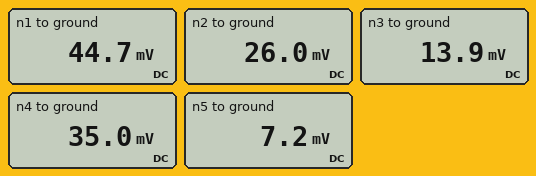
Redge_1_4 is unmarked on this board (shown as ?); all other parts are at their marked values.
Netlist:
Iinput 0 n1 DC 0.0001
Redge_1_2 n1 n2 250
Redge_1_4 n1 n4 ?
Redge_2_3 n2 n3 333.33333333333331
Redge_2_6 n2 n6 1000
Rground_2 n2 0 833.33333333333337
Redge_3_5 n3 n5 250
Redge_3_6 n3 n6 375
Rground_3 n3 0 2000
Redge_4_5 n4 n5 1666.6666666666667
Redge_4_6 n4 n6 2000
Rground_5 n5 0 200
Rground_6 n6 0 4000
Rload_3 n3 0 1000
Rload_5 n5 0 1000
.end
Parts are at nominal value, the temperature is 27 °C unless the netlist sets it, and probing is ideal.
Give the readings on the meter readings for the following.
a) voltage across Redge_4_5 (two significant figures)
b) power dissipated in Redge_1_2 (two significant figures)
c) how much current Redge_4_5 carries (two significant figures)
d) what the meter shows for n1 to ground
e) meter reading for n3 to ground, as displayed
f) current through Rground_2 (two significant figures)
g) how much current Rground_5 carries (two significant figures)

28 mV
1.4 µW
17 µA
44.7 mV
13.9 mV
31 µA
36 µA
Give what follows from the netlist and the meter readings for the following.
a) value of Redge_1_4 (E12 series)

390 Ω
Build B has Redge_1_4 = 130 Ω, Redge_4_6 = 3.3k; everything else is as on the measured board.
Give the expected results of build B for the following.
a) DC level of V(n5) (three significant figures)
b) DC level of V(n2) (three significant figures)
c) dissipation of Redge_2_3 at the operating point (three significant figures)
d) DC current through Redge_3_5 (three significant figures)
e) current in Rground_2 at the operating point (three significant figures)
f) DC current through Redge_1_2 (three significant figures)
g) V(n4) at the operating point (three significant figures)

7.44 mV
25.4 mV
411 nW
24.9 µA
30.5 µA
73.4 µA
40.3 mV
